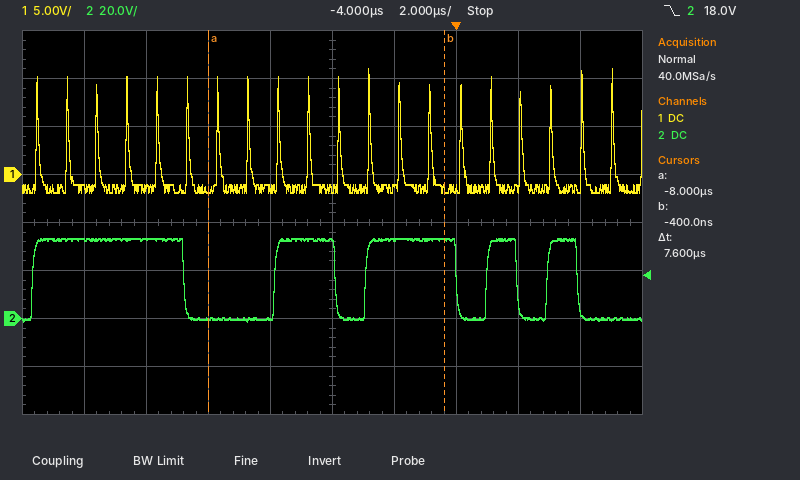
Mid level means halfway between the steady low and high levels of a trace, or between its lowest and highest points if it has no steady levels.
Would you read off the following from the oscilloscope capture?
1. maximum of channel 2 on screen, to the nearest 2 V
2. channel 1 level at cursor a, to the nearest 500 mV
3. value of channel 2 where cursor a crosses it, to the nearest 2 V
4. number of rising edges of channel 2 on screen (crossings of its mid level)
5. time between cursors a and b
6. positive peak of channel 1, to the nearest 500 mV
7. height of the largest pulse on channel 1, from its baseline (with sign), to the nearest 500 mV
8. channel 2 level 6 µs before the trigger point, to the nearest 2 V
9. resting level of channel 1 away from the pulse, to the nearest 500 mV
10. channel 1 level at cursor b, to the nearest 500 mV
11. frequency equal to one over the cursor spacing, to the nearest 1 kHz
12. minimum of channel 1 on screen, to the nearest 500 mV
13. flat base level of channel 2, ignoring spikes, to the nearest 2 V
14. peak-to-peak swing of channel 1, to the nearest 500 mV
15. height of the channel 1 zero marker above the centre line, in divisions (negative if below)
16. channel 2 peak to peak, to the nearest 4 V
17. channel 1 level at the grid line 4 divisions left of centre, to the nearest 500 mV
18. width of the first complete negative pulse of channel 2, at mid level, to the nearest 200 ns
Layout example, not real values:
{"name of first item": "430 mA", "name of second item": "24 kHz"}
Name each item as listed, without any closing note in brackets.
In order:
{"maximum of channel 2 on screen, to the nearest 2 V": "34 V", "channel 1 level at cursor a, to the nearest 500 mV": "-1.5 V", "value of channel 2 where cursor a crosses it, to the nearest 2 V": "0 V", "number of rising edges of channel 2 on screen": "5", "time between cursors a and b": "7.6 µs", "positive peak of channel 1, to the nearest 500 mV": "11.0 V", "height of the largest pulse on channel 1, from its baseline (with sign), to the nearest 500 mV": "+12.5 V", "channel 2 level 6 µs before the trigger point, to the nearest 2 V": "0 V", "resting level of channel 1 away from the pulse, to the nearest 500 mV": "-1.5 V", "channel 1 level at cursor b, to the nearest 500 mV": "-1.5 V", "frequency equal to one over the cursor spacing, to the nearest 1 kHz": "132 kHz", "minimum of channel 1 on screen, to the nearest 500 mV": "-2.0 V", "flat base level of channel 2, ignoring spikes, to the nearest 2 V": "0 V", "peak-to-peak swing of channel 1, to the nearest 500 mV": "13.0 V", "height of the channel 1 zero marker above the centre line, in divisions": "+1.0 div", "channel 2 peak to peak, to the nearest 4 V": "36 V", "channel 1 level at the grid line 4 divisions left of centre, to the nearest 500 mV": "-1.5 V", "width of the first complete negative pulse of channel 2, at mid level, to the nearest 200 ns": "3.0 µs"}
